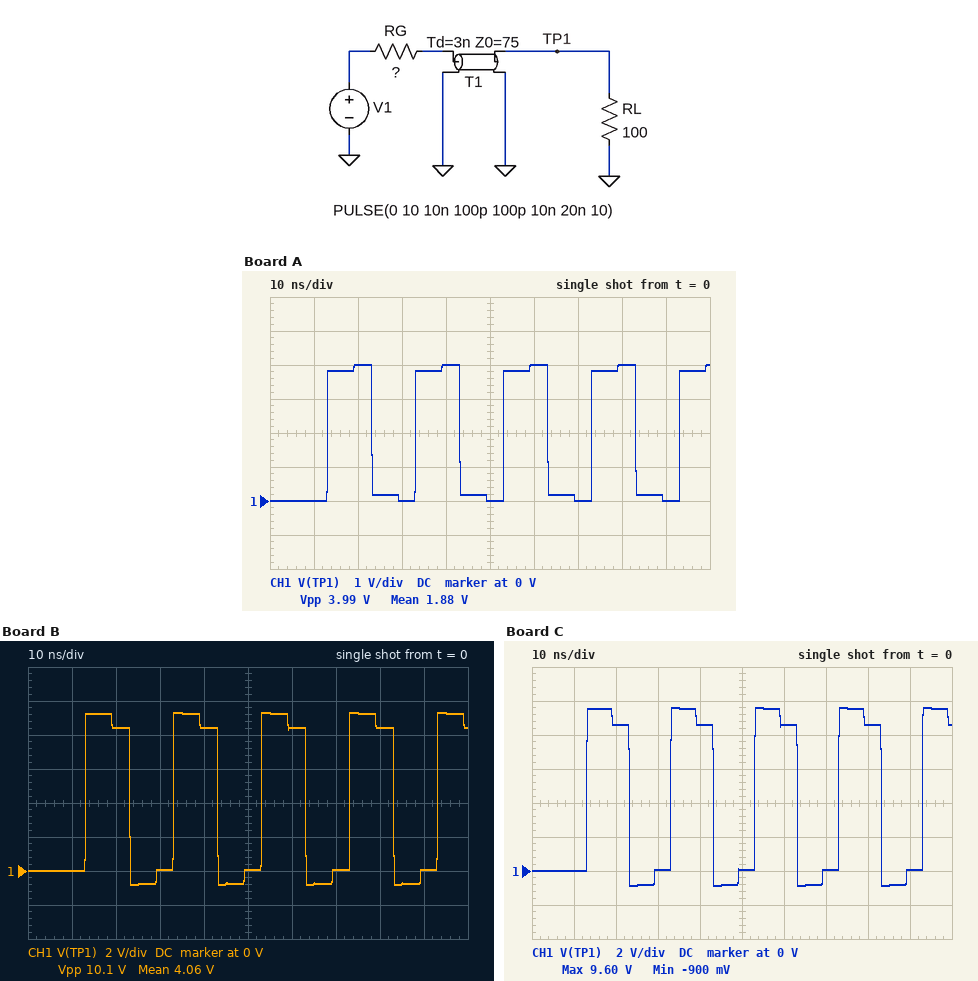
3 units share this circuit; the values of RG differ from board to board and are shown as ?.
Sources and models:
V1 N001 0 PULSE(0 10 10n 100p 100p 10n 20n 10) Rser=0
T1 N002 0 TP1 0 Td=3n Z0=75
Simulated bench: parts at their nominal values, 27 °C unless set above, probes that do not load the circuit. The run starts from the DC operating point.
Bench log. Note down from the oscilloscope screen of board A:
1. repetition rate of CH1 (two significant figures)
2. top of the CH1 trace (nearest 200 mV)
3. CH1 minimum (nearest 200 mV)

50 MHz
4.0 V
0 V
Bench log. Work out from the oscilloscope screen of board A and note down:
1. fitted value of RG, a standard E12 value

150 Ω
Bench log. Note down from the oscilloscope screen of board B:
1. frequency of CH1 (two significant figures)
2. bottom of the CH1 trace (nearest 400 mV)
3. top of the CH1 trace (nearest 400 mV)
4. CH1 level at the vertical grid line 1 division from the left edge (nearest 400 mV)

50 MHz
-800 mV
9.2 V
0 V
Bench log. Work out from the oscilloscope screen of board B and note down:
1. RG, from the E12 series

18 Ω
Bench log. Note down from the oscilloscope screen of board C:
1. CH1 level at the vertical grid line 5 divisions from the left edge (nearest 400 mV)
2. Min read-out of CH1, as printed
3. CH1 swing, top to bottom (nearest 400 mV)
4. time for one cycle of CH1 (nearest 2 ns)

0 V
-900 mV
10.4 V
20 ns
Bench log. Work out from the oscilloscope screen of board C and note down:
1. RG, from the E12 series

15 Ω
